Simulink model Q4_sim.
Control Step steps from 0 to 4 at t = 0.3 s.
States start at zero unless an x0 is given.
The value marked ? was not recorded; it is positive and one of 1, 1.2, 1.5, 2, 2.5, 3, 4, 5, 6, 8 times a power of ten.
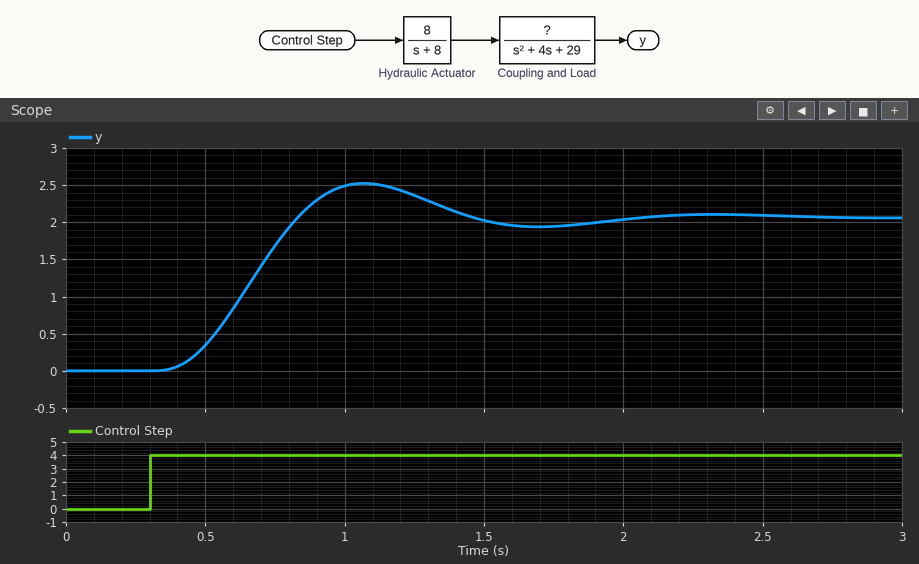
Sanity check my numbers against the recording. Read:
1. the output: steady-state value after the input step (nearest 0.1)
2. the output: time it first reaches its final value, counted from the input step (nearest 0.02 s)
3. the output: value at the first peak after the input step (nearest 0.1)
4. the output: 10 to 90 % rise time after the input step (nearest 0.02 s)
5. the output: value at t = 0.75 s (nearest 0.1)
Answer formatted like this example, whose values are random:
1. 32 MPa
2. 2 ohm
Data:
1. 2.1
2. 0.54 s
3. 2.5
4. 0.32 s
5. 1.7
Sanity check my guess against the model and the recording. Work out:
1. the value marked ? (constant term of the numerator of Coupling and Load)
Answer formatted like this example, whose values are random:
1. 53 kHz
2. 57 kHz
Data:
1. 15
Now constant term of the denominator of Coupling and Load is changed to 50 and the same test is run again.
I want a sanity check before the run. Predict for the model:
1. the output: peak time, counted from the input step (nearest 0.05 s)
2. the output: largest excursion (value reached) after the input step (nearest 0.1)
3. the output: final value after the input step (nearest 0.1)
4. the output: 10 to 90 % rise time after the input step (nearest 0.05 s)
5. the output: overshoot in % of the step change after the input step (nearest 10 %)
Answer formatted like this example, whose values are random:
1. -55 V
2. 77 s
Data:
1. 0.60 s
2. 1.5
3. 1.2
4. 0.25 s
5. 30 %
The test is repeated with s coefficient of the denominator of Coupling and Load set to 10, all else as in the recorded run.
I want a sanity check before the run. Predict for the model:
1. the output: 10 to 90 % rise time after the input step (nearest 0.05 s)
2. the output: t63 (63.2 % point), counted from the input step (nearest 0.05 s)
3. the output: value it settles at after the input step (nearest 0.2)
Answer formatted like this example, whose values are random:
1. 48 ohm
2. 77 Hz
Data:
1. 0.65 s
2. 0.50 s
3. 2.0
